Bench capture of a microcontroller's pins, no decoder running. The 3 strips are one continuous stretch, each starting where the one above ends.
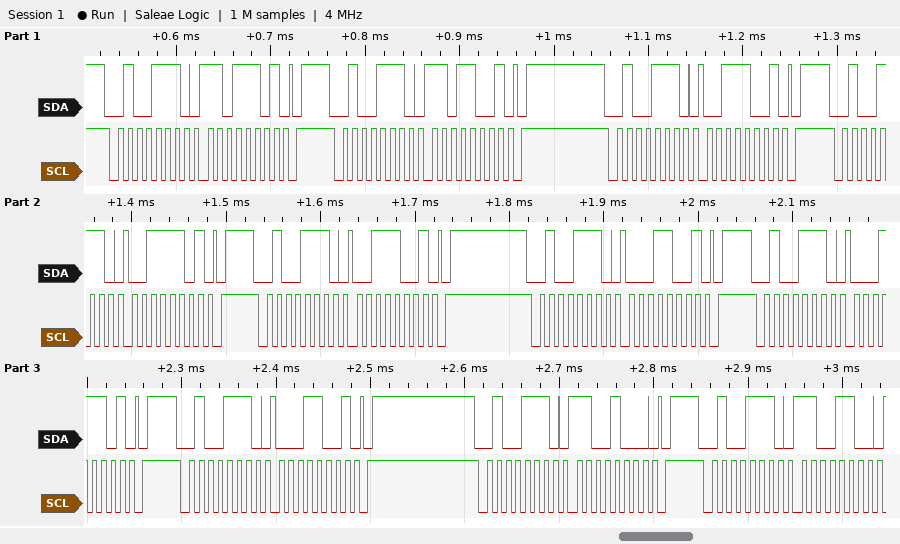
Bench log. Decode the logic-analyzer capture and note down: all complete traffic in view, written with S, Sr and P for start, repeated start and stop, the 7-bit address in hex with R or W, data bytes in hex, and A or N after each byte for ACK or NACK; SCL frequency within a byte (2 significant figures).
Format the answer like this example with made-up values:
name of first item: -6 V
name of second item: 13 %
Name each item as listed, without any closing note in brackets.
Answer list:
all complete traffic in view, written with S, Sr and P for start, repeated start and stop, the 7-bit address in hex with R or W, data bytes in hex, and A or N after each byte for ACK or NACK: S 27W A DD A P S 27W A D9 A P S 27W A 39 A P S 27W A 3D A P S 27W A 39 A P S 27W A 19 A P S 27W A 1D A P S 27W A 19 A P S 27W A C8 A P S 27W A CC A
SCL frequency within a byte: 100 kHz
